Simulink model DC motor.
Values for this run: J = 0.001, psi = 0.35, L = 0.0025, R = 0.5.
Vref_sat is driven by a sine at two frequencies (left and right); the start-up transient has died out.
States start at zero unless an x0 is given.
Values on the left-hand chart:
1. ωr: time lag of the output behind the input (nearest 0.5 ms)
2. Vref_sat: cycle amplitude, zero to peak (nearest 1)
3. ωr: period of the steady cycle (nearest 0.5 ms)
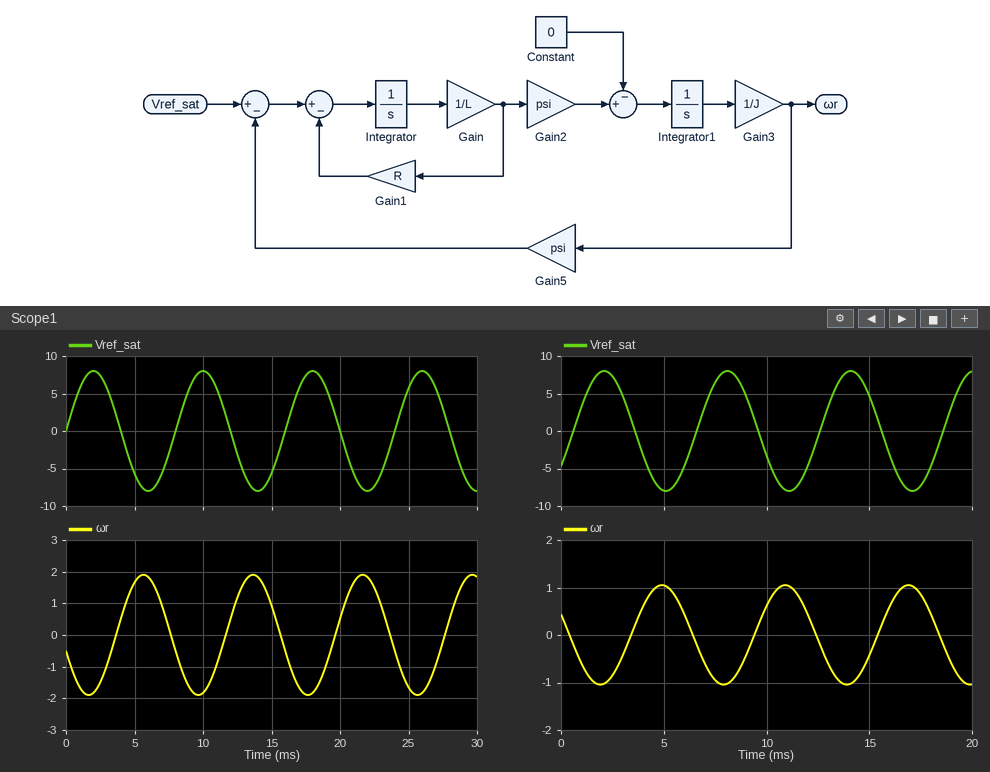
3.5 ms
8
8.0 ms
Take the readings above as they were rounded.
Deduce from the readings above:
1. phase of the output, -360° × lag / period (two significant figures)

-160°
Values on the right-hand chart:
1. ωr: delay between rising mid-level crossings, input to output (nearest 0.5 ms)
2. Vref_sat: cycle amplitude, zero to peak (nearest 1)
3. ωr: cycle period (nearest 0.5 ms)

3.0 ms
8
6.0 ms
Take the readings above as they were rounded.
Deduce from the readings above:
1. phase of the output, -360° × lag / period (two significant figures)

-180°
